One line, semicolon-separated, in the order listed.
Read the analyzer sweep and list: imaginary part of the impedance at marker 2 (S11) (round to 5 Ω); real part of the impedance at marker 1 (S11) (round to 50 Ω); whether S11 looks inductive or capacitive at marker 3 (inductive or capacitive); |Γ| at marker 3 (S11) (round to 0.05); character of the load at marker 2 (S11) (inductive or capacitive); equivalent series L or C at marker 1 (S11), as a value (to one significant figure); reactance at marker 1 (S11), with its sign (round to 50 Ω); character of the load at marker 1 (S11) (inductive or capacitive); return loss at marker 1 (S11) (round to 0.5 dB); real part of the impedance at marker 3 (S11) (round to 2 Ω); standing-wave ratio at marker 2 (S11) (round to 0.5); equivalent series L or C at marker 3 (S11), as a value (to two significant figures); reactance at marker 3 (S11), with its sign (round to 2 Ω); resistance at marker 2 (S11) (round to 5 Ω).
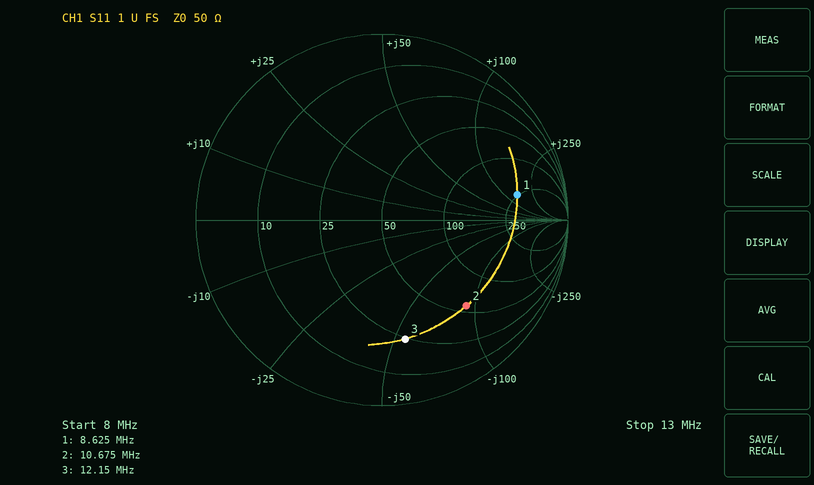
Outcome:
-90 Ω; 250 Ω; capacitive; 0.65; capacitive; 3 µH; +150 Ω; inductive; 2.5 dB; 24 Ω; 4.5; 240 pF; -54 Ω; 55 Ω
